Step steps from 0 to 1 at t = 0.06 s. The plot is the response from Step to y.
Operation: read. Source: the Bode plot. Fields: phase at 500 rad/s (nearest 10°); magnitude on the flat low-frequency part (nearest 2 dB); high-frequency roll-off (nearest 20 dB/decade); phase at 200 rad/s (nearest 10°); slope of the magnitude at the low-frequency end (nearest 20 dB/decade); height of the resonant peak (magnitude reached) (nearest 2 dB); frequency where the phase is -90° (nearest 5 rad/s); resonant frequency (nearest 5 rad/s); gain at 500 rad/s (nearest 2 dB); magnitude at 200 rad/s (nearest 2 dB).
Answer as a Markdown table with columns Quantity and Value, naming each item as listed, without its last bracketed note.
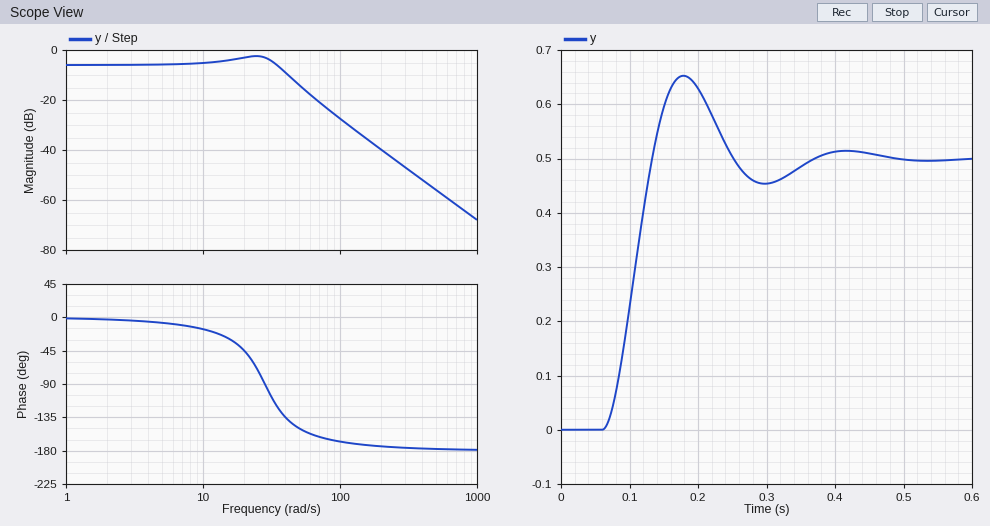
| Quantity | Value |
|---|---|
| phase at 500 rad/s | -180° |
| magnitude on the flat low-frequency part | -6 dB |
| high-frequency roll-off | -40 dB/decade |
| phase at 200 rad/s | -170° |
| slope of the magnitude at the low-frequency end | 0 dB/decade |
| height of the resonant peak (magnitude reached) | -2 dB |
| frequency where the phase is -90° | 30 rad/s |
| resonant frequency | 25 rad/s |
| gain at 500 rad/s | -56 dB |
| magnitude at 200 rad/s | -40 dB |
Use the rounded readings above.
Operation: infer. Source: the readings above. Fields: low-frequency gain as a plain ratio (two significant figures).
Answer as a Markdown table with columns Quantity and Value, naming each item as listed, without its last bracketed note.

| Quantity | Value |
|---|---|
| low-frequency gain as a plain ratio | 0.50 |
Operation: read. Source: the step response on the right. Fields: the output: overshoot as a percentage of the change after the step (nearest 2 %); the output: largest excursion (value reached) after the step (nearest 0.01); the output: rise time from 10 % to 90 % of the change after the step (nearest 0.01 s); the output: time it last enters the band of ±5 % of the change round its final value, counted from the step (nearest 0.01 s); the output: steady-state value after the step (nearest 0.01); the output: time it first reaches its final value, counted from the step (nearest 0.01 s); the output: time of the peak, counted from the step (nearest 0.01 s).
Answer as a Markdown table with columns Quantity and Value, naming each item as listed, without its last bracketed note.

| Quantity | Value |
|---|---|
| the output: overshoot as a percentage of the change after the step | 30 % |
| the output: largest excursion (value reached) after the step | 0.65 |
| the output: rise time from 10 % to 90 % of the change after the step | 0.05 s |
| the output: time it last enters the band of ±5 % of the change round its final value, counted from the step | 0.28 s |
| the output: steady-state value after the step | 0.50 |
| the output: time it first reaches its final value, counted from the step | 0.07 s |
| the output: time of the peak, counted from the step | 0.12 s |
